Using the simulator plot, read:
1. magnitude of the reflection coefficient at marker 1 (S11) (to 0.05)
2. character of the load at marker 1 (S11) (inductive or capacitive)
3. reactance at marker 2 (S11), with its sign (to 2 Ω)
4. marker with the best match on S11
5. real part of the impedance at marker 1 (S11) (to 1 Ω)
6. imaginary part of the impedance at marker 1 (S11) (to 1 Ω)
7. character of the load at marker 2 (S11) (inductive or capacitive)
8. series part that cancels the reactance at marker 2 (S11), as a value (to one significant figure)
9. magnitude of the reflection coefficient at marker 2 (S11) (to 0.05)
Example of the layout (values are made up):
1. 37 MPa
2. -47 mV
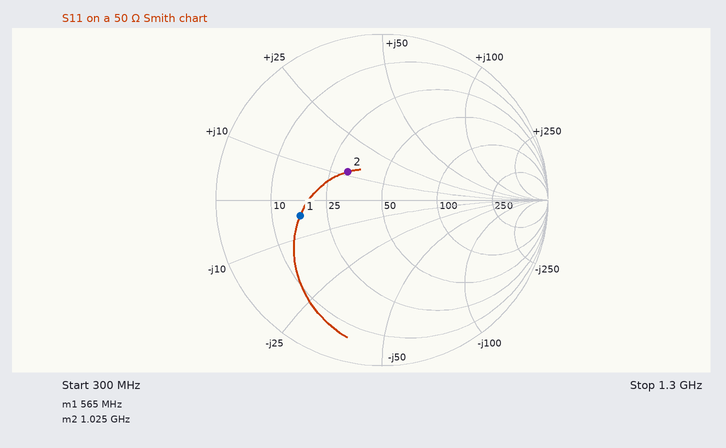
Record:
1. 0.50
2. capacitive
3. +12 Ω
4. marker 2
5. 17 Ω
6. -4 Ω
7. inductive
8. 10 pF
9. 0.25
